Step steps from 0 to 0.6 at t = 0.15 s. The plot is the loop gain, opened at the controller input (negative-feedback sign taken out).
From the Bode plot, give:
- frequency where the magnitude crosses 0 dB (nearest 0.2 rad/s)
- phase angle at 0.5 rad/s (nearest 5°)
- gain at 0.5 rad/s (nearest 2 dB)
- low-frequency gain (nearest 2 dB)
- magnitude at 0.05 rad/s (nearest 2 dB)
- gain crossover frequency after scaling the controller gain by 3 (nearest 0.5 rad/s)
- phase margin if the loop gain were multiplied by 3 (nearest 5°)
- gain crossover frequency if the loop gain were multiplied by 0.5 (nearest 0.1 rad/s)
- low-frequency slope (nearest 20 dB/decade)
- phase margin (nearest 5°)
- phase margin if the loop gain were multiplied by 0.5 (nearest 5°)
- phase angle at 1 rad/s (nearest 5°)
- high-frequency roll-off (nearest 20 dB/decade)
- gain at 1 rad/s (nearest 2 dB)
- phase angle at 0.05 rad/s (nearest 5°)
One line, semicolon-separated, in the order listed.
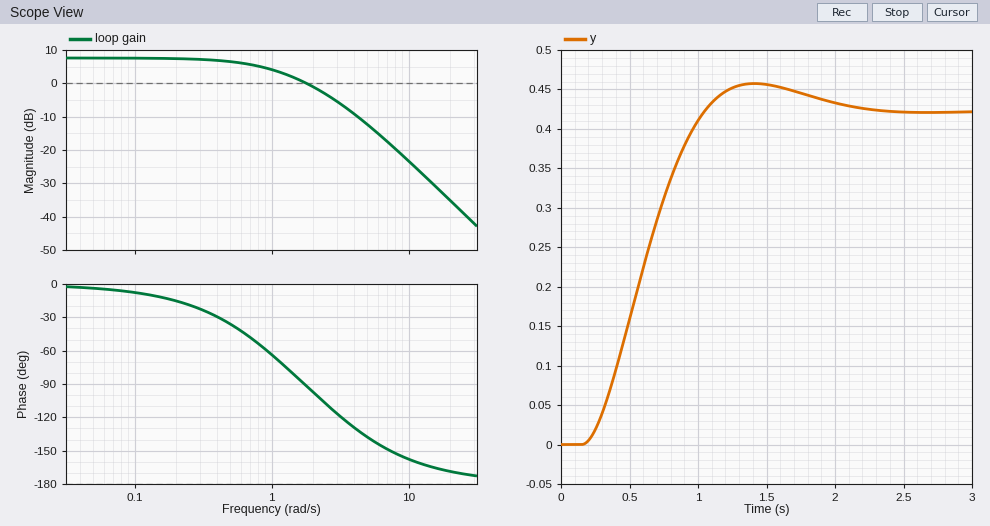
1.8 rad/s; -35°; 6 dB; 8 dB; 8 dB; 4.0 rad/s; 50°; 0.6 rad/s; 0 dB/decade; 90°; 135°; -65°; -40 dB/decade; 4 dB; -5°
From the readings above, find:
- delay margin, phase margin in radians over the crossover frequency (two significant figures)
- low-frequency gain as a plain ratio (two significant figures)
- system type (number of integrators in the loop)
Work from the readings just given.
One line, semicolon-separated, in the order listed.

0.87 s; 2.5; 0
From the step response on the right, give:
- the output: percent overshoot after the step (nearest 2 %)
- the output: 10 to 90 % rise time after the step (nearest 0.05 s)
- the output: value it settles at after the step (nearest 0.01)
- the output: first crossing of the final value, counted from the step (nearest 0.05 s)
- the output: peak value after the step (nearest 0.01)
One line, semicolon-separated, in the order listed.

8 %; 0.60 s; 0.42; 0.90 s; 0.46
